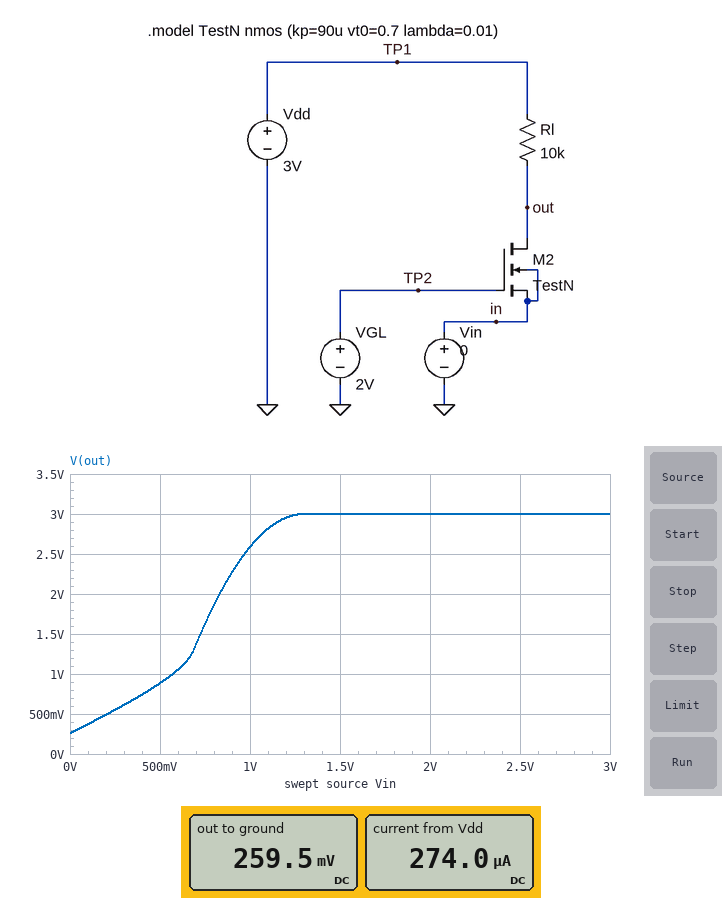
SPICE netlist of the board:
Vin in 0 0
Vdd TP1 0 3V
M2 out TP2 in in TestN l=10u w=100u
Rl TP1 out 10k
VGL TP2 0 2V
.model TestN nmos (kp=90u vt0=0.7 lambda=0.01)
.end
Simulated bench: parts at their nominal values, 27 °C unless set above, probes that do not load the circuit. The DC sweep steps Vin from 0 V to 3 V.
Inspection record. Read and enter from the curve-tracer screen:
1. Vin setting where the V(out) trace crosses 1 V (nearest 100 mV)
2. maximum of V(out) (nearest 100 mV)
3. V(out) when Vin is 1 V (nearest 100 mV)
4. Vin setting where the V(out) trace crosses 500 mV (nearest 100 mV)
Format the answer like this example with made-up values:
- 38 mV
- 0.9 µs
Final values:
- 600 mV
- 3.0 V
- 2.6 V
- 200 mV
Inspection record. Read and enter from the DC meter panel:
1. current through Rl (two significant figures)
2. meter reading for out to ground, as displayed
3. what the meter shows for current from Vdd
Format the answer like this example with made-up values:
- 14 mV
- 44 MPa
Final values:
- 270 µA
- 259.5 mV
- 274.0 µA
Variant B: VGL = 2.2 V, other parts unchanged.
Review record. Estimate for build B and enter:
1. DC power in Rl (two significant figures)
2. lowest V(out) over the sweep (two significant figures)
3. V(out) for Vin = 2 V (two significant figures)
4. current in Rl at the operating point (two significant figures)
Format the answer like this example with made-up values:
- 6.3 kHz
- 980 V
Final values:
- 770 µW
- 220 mV
- 3.0 V
- 280 µA
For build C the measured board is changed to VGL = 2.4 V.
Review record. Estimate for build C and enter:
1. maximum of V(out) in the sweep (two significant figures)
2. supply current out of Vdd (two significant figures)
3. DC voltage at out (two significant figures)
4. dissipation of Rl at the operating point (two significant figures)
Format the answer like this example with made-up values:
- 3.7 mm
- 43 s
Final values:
- 3.0 V
- 280 µA
- 190 mV
- 790 µW
